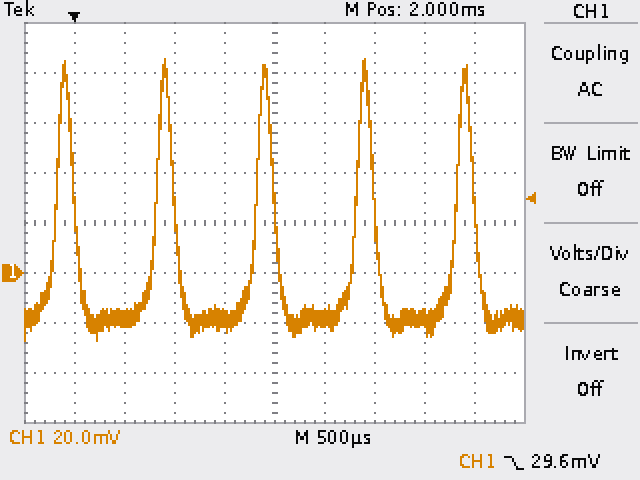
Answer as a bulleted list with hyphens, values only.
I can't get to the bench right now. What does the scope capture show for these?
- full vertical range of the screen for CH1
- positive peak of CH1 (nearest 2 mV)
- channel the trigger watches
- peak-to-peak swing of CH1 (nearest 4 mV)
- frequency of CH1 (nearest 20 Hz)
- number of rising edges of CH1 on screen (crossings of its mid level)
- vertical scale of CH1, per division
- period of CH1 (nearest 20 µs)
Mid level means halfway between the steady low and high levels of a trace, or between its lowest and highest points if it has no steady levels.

- 160 mV
- 86 mV
- CH1
- 112 mV
- 1.00 kHz
- 5
- 20 mV
- 1.00 ms
